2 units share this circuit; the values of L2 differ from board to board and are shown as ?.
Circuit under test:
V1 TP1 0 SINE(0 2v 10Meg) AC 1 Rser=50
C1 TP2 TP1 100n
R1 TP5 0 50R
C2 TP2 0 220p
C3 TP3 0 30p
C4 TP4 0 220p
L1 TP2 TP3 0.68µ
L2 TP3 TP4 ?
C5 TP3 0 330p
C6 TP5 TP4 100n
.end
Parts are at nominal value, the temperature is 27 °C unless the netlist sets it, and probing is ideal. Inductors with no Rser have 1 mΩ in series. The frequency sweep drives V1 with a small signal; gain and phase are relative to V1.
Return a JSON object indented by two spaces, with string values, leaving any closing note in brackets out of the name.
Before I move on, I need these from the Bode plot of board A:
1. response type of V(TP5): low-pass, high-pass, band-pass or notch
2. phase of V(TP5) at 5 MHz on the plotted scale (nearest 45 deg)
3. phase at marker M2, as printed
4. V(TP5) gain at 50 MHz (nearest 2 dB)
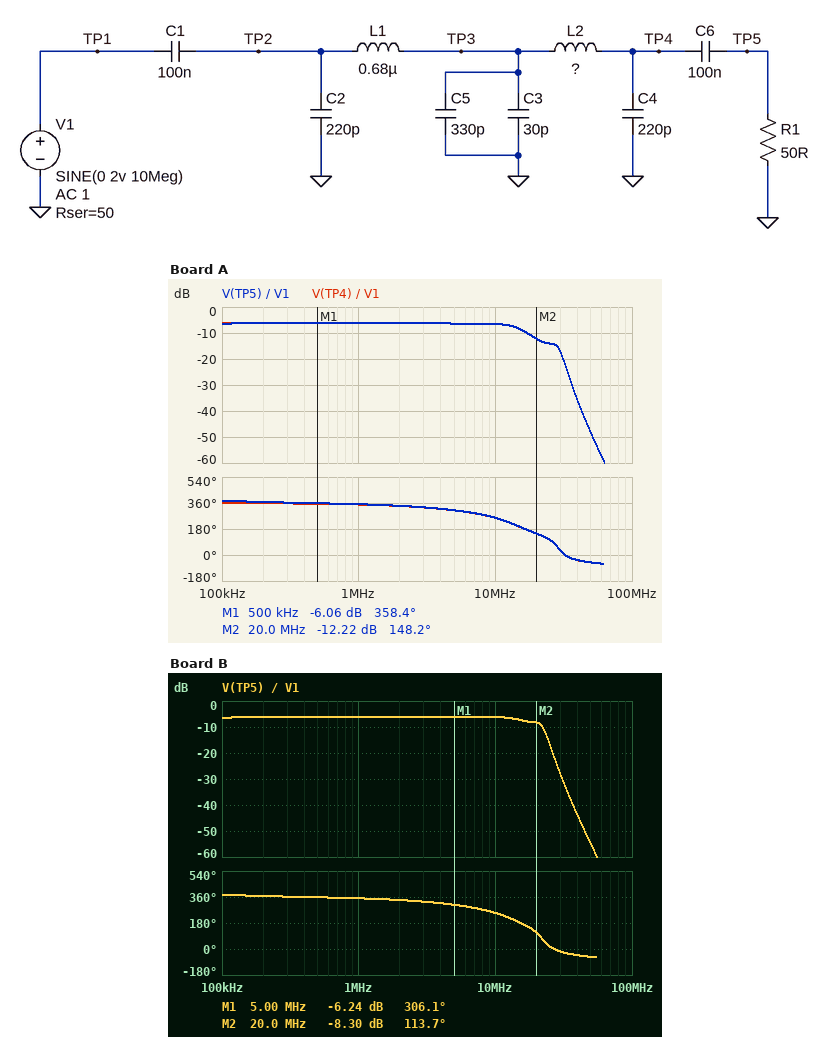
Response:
{
  "response type of V(TP5): low-pass, high-pass, band-pass or notch": "low-pass",
  "phase of V(TP5) at 5 MHz on the plotted scale": "315 deg",
  "phase at marker M2, as printed": "148.2 deg",
  "V(TP5) gain at 50 MHz": "-48 dB"
}
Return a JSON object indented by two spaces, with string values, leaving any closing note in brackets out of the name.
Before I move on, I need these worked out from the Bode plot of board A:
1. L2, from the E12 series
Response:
{
  "L2, from the E12 series": "220 nH"
}
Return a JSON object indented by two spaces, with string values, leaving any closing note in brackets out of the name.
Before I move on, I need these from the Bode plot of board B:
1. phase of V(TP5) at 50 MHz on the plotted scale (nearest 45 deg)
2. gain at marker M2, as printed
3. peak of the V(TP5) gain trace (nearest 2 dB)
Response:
{
  "phase of V(TP5) at 50 MHz on the plotted scale": "-45 deg",
  "gain at marker M2, as printed": "-8.30 dB",
  "peak of the V(TP5) gain trace": "-6 dB"
}
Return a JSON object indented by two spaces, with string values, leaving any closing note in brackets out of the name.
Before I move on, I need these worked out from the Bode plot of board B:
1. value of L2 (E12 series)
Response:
{
  "value of L2": "390 nH"
}
